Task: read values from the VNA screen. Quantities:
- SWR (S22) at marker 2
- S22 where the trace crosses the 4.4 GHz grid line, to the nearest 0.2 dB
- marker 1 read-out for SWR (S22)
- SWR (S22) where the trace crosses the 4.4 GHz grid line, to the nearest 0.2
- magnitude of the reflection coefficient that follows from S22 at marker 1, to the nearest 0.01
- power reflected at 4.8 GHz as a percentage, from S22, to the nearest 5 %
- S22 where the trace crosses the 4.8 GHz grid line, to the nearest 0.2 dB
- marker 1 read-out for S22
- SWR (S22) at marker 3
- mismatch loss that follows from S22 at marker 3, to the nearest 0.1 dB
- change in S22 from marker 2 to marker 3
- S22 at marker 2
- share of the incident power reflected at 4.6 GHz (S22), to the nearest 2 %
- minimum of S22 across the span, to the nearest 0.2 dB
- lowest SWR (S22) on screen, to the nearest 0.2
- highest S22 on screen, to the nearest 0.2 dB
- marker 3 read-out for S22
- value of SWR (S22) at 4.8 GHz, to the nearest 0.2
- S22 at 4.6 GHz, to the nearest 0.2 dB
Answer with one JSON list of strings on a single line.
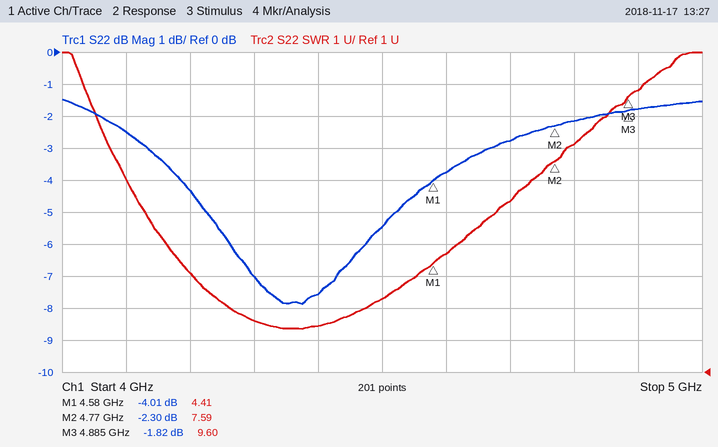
["7.59", "-7.6 dB", "4.41", "2.4", "0.63", "60 %", "-2.2 dB", "-4.01 dB", "9.60", "4.7 dB", "0.48 dB", "-2.30 dB", "42 %", "-7.8 dB", "2.4", "-1.4 dB", "-1.82 dB", "8.2", "-3.8 dB"]
